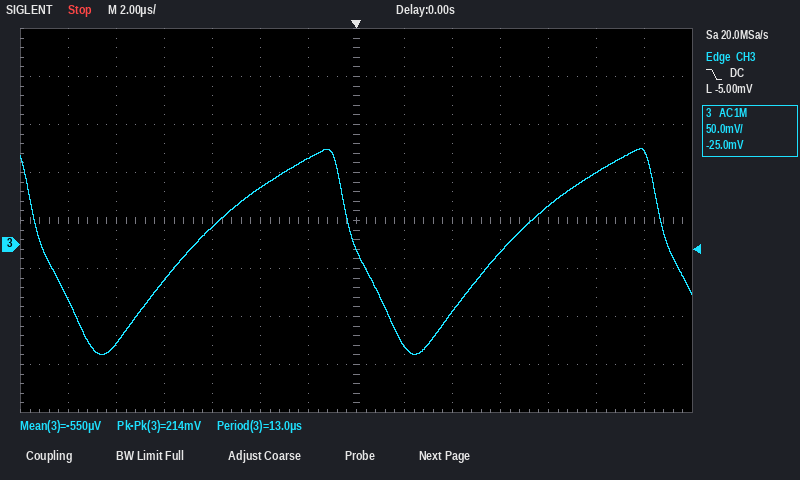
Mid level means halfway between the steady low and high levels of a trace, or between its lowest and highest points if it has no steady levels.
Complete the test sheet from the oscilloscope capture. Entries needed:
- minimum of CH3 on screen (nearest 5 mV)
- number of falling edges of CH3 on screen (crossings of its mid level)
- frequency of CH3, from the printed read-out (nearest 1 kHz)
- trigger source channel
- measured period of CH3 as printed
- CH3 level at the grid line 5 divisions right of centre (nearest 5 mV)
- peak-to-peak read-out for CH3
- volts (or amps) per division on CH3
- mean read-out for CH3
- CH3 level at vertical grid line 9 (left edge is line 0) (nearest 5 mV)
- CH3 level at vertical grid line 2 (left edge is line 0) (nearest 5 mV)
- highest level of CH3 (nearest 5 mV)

-115 mV
3
77 kHz
CH3
13.0 µs
75 mV
214 mV
50 mV
-550 µV
-70 mV
-105 mV
100 mV
